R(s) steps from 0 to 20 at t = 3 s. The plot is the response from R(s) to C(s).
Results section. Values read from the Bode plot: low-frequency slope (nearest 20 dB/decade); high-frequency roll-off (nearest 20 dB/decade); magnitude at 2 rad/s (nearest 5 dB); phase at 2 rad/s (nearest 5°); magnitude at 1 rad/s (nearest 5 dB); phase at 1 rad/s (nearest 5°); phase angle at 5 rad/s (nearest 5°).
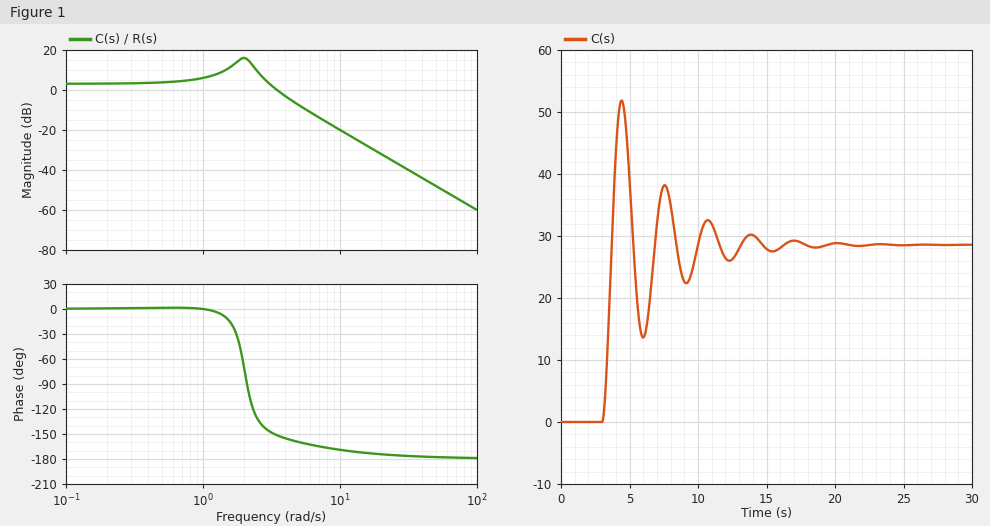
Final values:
0 dB/decade
-40 dB/decade
15 dB
-70°
5 dB
0°
-160°
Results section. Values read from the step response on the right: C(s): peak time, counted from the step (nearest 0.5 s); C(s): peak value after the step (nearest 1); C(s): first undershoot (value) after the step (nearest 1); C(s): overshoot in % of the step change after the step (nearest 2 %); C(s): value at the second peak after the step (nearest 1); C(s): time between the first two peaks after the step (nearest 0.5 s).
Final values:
1.5 s
52
14
82 %
38
3.0 s
